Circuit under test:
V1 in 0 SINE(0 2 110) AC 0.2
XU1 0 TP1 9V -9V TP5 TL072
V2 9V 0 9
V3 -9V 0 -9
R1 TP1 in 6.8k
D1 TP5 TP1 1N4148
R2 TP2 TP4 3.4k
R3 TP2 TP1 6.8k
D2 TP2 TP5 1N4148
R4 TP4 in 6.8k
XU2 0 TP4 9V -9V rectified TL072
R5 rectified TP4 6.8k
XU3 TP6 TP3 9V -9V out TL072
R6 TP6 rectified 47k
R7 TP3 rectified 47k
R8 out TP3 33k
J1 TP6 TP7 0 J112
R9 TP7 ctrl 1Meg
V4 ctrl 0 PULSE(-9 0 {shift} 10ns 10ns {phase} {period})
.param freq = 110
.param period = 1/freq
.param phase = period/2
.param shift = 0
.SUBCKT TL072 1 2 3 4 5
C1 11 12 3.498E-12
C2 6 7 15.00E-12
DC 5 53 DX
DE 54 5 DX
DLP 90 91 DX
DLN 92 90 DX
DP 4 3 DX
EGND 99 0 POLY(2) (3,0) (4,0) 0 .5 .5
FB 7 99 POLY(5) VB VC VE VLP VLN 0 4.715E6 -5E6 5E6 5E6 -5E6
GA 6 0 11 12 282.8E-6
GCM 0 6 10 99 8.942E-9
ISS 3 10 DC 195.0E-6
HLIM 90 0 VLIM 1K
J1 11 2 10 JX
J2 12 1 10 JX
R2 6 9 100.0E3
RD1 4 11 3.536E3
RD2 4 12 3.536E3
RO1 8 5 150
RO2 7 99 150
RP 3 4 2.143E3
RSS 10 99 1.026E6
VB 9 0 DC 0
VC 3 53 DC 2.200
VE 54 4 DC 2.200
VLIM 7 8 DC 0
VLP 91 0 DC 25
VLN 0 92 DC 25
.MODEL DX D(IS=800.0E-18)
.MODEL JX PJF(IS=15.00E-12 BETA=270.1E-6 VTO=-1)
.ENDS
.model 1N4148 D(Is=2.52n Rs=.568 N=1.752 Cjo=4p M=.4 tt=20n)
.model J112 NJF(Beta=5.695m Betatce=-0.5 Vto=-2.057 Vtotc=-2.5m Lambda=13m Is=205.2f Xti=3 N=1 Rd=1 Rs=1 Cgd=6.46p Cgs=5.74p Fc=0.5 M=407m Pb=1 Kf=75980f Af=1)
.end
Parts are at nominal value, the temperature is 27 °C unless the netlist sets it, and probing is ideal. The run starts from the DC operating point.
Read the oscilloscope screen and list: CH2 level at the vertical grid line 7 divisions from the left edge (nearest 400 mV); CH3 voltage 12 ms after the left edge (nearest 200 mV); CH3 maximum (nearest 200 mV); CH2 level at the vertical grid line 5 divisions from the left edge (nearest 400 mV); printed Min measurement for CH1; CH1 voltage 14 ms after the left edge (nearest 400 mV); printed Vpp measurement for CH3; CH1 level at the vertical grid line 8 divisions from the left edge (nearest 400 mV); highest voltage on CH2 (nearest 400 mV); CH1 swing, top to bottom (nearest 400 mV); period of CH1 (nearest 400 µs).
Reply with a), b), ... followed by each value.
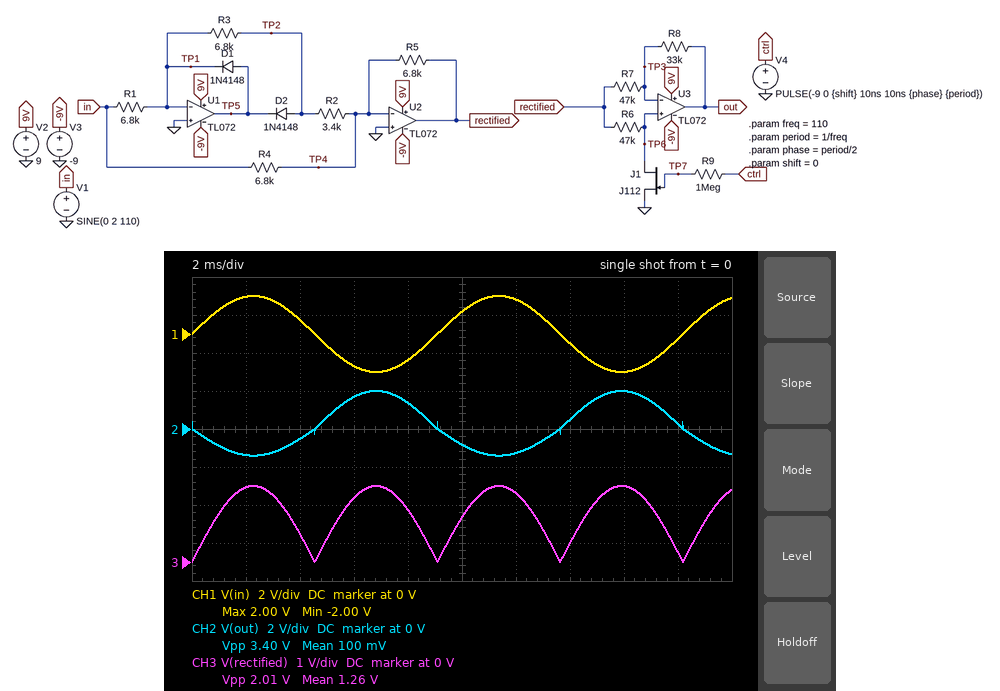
a) 400 mV
b) 1.8 V
c) 2.0 V
d) -800 mV
e) -2.00 V
f) -400 mV
g) 2.01 V
h) -2.0 V
i) 2.0 V
j) 4.0 V
k) 9.2 ms
